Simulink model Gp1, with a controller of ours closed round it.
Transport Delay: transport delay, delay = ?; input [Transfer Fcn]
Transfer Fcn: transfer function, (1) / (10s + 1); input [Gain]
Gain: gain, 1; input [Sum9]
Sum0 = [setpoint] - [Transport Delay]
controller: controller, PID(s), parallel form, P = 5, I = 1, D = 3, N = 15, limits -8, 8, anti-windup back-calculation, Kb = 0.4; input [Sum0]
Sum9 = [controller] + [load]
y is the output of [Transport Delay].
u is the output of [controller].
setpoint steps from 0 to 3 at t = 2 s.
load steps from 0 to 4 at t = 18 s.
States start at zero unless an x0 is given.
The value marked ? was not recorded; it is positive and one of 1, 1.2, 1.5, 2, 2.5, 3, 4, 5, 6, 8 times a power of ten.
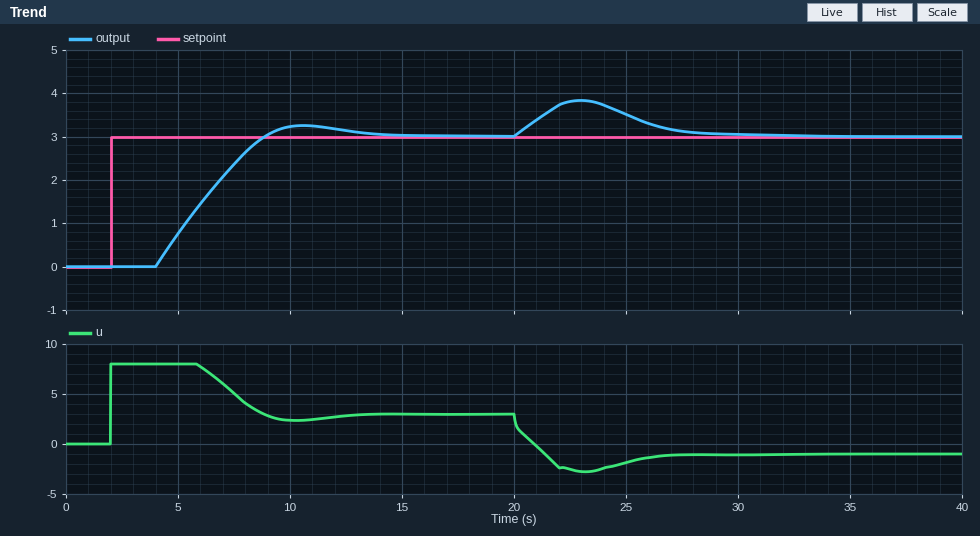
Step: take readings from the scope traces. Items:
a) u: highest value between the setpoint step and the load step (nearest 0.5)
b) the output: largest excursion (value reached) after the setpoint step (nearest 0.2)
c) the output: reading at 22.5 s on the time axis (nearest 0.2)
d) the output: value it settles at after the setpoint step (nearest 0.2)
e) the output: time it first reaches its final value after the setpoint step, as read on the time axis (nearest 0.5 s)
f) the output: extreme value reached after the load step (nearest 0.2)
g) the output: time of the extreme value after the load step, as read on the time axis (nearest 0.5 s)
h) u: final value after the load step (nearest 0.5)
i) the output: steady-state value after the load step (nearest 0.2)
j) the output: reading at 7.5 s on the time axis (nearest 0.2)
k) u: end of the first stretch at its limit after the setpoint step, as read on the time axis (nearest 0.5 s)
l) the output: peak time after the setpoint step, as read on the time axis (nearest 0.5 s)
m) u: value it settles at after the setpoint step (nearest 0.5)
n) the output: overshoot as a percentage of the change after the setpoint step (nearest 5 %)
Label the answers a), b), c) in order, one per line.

a) 8.0
b) 3.2
c) 3.8
d) 3.0
e) 9.0 s
f) 3.8
g) 23.0 s
h) -1.0
i) 3.0
j) 2.4
k) 6.0 s
l) 10.5 s
m) 3.0
n) 10 %
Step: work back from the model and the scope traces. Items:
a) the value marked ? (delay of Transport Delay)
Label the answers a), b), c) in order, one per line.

a) 2
